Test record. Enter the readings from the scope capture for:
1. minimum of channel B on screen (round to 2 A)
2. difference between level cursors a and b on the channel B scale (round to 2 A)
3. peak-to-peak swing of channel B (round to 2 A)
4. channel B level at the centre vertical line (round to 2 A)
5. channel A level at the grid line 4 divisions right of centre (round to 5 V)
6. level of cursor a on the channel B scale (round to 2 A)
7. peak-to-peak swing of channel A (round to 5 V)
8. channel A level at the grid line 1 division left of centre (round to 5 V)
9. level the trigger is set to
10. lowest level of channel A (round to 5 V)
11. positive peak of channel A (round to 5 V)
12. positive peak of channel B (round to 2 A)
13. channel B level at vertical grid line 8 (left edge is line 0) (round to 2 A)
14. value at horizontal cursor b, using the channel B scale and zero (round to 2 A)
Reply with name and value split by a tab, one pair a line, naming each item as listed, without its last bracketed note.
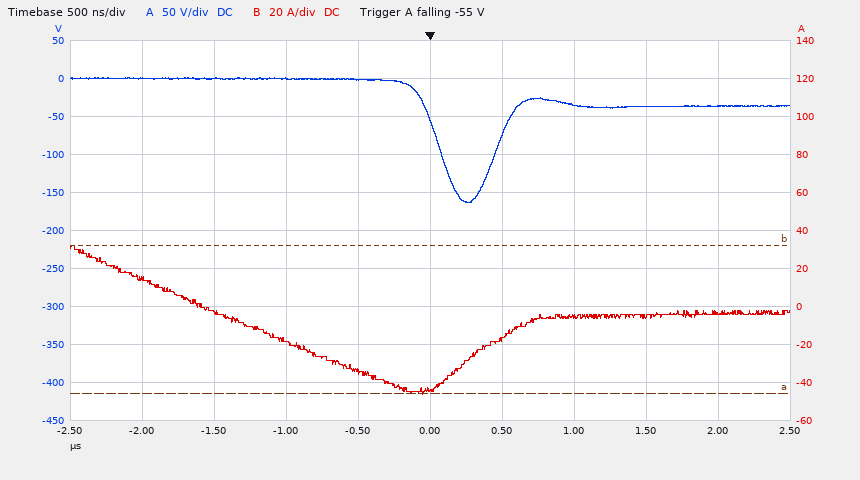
minimum of channel B on screen	-46 A
difference between level cursors a and b on the channel B scale	78 A
peak-to-peak swing of channel B	78 A
channel B level at the centre vertical line	-44 A
channel A level at the grid line 4 divisions right of centre	-35 V
level of cursor a on the channel B scale	-46 A
peak-to-peak swing of channel A	165 V
channel A level at the grid line 1 division left of centre	0 V
level the trigger is set to	-55 V
lowest level of channel A	-165 V
positive peak of channel A	0 V
positive peak of channel B	32 A
channel B level at vertical grid line 8 (left edge is line 0)	-6 A
value at horizontal cursor b, using the channel B scale and zero	32 A
